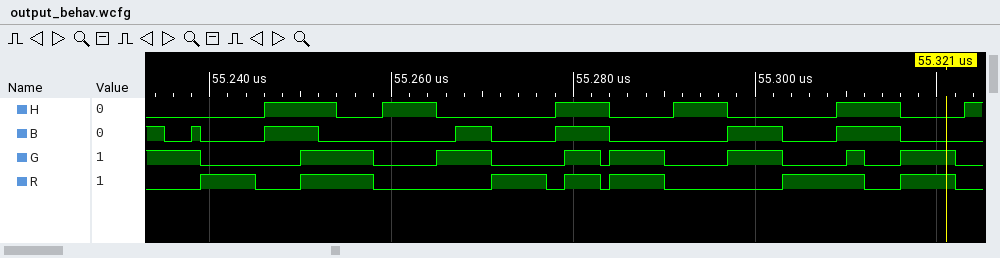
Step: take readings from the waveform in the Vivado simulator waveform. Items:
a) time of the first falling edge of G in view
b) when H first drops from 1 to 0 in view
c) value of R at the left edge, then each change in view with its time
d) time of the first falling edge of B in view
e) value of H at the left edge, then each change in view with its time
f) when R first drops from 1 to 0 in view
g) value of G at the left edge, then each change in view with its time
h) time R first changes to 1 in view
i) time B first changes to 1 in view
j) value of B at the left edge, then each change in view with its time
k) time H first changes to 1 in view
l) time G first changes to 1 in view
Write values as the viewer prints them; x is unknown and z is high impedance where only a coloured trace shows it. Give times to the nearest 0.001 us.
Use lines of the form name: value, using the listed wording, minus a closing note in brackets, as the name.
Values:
time of the first falling edge of G in view: 55.239 us
when H first drops from 1 to 0 in view: 55.254 us
value of R at the left edge, then each change in view with its time: 0, 1 at 55.239 us, 0 at 55.245 us, 1 at 55.25 us, 0 at 55.258 us, 1 at 55.271 us, 0 at 55.277 us, 1 at 55.279 us, 0 at 55.283 us, 1 at 55.284 us, 0 at 55.29 us, 1 at 55.303 us, 0 at 55.312 us, 1 at 55.316 us, 0 at 55.322 us
time of the first falling edge of B in view: 55.235 us
value of H at the left edge, then each change in view with its time: 0, 1 at 55.246 us, 0 at 55.254 us, 1 at 55.259 us, 0 at 55.265 us, 1 at 55.278 us, 0 at 55.284 us, 1 at 55.291 us, 0 at 55.297 us, 1 at 55.309 us, 0 at 55.316 us, 1 at 55.323 us
when R first drops from 1 to 0 in view: 55.245 us
value of G at the left edge, then each change in view with its time: 1, 0 at 55.239 us, 1 at 55.25 us, 0 at 55.258 us, 1 at 55.265 us, 0 at 55.271 us, 1 at 55.279 us, 0 at 55.283 us, 1 at 55.284 us, 0 at 55.29 us, 1 at 55.297 us, 0 at 55.303 us, 1 at 55.31 us, 0 at 55.312 us, 1 at 55.316 us, 0 at 55.322 us
time R first changes to 1 in view: 55.239 us
time B first changes to 1 in view: 55.238 us
value of B at the left edge, then each change in view with its time: 1, 0 at 55.235 us, 1 at 55.238 us, 0 at 55.239 us, 1 at 55.246 us, 0 at 55.252 us, 1 at 55.267 us, 0 at 55.271 us, 1 at 55.278 us, 0 at 55.284 us, 1 at 55.297 us, 0 at 55.303 us, 1 at 55.309 us, 0 at 55.316 us
time H first changes to 1 in view: 55.246 us
time G first changes to 1 in view: 55.25 us
